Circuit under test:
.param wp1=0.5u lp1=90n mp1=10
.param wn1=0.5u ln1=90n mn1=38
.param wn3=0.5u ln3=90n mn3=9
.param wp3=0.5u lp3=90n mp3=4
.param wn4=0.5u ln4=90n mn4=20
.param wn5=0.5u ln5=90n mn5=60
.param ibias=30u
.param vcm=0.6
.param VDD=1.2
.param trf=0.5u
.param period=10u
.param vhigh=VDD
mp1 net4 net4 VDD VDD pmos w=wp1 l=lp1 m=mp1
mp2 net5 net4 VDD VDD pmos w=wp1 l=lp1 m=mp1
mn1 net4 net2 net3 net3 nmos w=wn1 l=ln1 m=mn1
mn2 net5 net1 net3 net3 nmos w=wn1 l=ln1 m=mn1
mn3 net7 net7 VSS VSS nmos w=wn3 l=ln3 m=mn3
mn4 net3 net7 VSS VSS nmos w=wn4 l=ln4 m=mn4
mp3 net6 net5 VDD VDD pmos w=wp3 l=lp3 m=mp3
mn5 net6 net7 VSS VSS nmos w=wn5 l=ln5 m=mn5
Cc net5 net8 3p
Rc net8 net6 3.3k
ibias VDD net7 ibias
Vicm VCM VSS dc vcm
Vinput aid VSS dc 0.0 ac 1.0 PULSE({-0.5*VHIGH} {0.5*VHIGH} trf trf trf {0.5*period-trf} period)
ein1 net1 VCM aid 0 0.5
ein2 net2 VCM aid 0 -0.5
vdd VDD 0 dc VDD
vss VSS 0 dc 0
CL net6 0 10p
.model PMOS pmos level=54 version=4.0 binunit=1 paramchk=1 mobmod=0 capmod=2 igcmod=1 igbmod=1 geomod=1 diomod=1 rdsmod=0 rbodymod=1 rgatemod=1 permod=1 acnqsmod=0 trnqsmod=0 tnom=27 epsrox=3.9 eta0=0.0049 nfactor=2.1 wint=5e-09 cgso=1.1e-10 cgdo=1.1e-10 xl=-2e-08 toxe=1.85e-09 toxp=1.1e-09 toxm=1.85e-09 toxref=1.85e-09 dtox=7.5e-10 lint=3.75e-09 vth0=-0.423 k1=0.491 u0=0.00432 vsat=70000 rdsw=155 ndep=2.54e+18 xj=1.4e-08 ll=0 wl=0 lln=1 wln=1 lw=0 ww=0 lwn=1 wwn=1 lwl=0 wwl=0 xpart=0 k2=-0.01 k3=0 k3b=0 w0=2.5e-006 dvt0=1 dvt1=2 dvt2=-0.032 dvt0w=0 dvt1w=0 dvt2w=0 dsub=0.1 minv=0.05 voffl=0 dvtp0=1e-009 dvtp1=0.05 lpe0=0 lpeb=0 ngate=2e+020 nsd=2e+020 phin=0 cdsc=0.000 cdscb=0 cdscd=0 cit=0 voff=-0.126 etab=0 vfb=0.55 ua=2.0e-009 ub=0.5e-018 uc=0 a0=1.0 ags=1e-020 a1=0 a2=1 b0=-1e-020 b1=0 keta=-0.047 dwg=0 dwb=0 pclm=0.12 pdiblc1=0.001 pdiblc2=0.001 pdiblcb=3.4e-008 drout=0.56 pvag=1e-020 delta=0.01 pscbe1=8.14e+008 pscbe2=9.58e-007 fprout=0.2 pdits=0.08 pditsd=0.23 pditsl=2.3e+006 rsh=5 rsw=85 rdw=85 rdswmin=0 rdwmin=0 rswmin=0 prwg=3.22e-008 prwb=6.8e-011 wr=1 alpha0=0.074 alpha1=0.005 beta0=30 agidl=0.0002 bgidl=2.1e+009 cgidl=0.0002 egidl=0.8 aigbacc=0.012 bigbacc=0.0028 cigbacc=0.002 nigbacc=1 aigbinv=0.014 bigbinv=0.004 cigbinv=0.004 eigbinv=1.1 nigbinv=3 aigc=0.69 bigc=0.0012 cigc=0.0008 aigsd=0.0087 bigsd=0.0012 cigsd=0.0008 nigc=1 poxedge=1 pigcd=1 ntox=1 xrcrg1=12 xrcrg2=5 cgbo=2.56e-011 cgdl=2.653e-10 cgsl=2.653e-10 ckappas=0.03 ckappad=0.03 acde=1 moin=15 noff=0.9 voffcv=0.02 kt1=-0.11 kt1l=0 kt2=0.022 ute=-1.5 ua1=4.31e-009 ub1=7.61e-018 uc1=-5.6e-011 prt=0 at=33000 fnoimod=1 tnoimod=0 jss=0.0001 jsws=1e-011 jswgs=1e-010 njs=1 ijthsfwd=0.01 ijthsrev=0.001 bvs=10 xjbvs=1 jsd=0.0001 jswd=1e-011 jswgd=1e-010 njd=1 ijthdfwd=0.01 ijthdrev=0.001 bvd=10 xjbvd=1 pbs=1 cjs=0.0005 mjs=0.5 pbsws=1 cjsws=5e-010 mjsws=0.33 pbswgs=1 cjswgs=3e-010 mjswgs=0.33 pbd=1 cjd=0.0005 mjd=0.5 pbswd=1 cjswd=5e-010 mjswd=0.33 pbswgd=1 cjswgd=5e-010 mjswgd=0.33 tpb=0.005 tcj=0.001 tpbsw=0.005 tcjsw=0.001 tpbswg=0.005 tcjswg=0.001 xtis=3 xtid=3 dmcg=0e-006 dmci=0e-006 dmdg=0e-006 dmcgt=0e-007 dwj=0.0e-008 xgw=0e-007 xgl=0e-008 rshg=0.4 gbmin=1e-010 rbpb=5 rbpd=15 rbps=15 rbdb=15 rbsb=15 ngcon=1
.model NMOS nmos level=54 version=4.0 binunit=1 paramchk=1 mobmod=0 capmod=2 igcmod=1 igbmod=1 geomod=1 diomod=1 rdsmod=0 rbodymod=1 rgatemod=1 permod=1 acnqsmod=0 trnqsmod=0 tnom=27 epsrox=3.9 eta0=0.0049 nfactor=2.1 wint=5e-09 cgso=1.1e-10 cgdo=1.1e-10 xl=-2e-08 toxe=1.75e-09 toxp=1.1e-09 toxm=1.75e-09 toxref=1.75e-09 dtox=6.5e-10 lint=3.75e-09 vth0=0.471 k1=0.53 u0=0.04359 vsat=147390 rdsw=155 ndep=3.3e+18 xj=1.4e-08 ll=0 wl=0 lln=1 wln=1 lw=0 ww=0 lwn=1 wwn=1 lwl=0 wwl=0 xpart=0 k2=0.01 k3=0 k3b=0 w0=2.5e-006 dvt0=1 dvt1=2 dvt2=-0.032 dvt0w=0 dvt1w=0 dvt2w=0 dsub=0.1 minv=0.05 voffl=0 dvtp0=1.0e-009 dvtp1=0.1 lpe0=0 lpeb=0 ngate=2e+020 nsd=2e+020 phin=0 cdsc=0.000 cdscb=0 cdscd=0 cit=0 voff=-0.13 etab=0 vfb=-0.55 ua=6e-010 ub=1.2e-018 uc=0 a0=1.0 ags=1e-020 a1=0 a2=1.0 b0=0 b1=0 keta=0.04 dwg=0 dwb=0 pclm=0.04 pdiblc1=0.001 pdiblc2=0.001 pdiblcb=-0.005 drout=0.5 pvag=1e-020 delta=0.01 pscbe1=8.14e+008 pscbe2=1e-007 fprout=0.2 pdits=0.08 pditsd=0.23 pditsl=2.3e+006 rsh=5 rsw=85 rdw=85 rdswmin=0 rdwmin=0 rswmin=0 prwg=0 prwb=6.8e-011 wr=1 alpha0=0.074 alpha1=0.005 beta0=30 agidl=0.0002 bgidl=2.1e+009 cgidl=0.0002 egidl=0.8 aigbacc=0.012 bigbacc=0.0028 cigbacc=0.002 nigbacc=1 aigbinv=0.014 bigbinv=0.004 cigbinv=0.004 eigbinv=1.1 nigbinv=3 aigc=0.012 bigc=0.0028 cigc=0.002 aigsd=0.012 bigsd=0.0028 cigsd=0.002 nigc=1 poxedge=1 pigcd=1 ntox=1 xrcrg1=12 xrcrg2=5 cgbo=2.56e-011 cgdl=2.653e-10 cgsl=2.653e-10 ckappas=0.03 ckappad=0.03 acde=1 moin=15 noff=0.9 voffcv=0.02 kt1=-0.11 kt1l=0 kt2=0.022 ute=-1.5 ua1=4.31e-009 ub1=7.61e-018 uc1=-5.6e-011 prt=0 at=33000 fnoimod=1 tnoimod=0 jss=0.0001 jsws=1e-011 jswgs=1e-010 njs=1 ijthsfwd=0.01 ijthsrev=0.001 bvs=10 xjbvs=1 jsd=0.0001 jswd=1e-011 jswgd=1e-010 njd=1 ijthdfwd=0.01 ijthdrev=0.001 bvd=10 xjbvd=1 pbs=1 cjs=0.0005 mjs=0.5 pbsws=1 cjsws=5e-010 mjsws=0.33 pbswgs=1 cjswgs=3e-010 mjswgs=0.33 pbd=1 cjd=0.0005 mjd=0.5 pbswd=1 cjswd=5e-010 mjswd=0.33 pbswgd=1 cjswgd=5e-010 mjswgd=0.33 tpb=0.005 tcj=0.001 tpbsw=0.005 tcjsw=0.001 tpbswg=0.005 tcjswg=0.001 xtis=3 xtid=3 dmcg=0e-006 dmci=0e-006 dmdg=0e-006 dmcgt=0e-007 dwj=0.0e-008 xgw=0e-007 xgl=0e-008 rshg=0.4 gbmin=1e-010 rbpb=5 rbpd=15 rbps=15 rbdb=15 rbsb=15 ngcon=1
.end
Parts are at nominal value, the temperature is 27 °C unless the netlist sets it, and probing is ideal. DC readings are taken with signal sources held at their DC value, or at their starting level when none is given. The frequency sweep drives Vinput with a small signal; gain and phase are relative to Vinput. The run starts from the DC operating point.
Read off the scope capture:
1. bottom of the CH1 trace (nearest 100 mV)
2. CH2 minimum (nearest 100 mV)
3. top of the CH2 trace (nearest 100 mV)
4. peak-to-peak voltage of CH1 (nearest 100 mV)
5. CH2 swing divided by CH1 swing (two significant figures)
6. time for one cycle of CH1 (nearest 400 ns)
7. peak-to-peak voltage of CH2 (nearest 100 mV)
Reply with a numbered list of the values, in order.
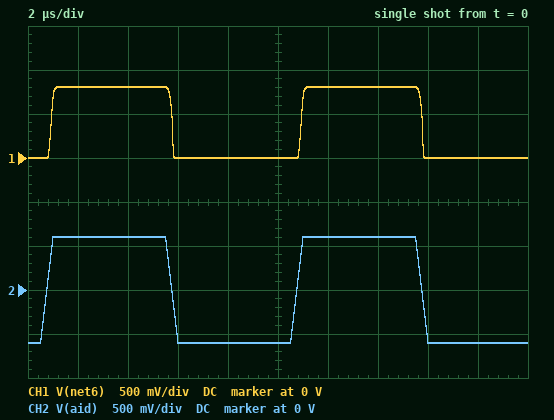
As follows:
1. 0 V
2. -600 mV
3. 600 mV
4. 800 mV
5. 1.5
6. 10.0 µs
7. 1.2 V
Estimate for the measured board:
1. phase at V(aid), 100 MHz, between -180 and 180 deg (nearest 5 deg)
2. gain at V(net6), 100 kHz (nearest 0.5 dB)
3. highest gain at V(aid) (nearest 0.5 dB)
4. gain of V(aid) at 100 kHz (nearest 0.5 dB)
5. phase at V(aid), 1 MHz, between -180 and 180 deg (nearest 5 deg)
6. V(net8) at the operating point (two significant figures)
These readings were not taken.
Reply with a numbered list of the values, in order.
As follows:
1. 0 deg
2. 1.5 dB
3. 0 dB
4. 0 dB
5. 0 deg
6. 3.0 mV
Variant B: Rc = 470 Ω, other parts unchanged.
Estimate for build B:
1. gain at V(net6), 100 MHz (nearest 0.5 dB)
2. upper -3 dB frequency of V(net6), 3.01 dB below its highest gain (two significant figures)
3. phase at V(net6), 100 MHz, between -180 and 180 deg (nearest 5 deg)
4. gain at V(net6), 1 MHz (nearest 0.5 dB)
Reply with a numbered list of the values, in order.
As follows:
1. -23.0 dB
2. 980 kHz
3. 135 deg
4. -1.5 dB
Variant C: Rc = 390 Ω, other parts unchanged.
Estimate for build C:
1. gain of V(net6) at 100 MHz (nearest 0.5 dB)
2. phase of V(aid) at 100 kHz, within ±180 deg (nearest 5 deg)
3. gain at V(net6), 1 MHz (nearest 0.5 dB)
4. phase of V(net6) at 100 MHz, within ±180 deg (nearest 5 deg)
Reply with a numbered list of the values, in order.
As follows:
1. -23.0 dB
2. 0 deg
3. -1.5 dB
4. 135 deg
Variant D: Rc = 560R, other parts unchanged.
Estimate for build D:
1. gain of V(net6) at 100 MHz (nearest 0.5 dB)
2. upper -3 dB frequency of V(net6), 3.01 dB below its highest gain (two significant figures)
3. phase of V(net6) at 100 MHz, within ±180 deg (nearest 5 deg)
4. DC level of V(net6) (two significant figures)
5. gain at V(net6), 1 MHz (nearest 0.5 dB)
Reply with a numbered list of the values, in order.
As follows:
1. -23.5 dB
2. 980 kHz
3. 135 deg
4. 3.0 mV
5. -1.5 dB
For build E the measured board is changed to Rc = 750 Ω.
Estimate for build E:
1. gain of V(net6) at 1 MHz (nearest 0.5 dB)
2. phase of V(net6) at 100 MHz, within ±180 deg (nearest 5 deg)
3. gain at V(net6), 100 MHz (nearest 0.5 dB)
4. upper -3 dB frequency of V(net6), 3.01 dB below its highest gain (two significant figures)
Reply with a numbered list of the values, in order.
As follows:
1. -1.5 dB
2. 135 deg
3. -23.5 dB
4. 980 kHz
